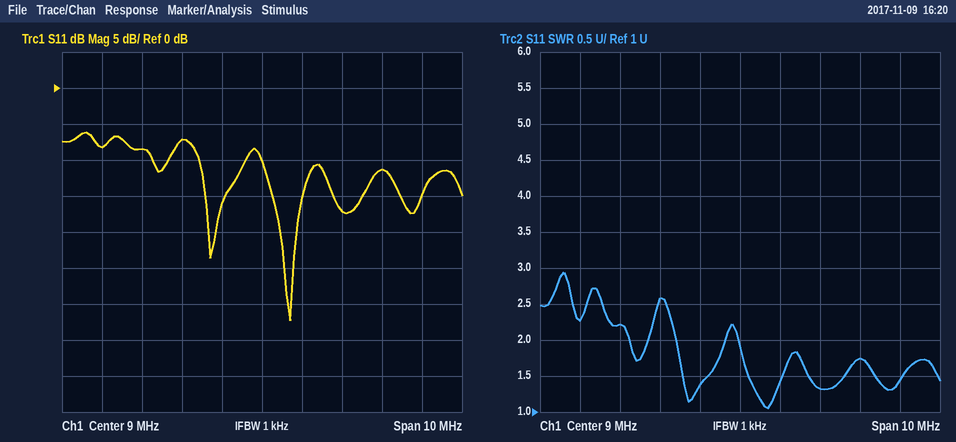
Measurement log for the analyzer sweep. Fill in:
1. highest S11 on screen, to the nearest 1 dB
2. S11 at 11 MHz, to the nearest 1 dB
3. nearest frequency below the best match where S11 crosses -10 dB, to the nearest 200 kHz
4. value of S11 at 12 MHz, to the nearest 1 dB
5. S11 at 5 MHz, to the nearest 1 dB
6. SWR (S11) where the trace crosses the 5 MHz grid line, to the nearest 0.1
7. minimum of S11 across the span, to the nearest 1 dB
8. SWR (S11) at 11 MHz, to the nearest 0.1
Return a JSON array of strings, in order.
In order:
["-6 dB", "-17 dB", "9.0 MHz", "-11 dB", "-8 dB", "2.3", "-32 dB", "1.3"]
